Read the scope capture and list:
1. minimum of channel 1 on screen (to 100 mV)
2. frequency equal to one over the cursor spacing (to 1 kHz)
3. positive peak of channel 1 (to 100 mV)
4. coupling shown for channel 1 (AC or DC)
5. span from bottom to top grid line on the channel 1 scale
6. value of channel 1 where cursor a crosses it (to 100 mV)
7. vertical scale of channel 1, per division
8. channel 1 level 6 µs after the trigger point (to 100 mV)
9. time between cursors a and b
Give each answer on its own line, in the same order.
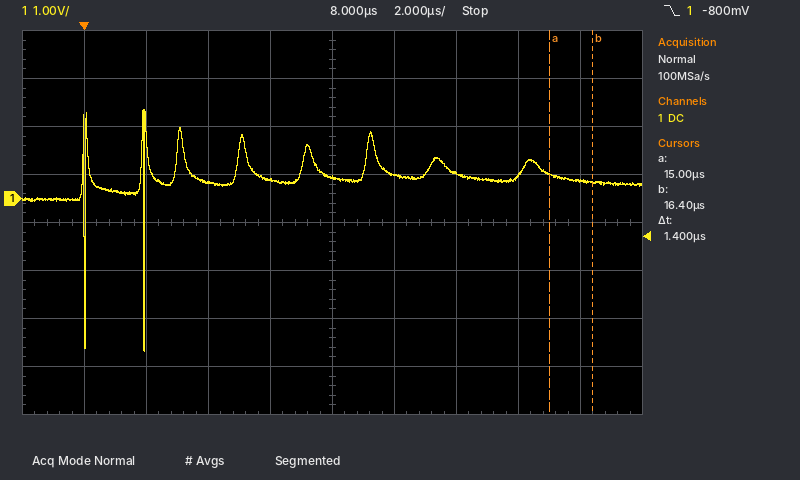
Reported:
-3.2 V
714 kHz
1.9 V
DC
8 V
500 mV
1 V
400 mV
1.4 µs
